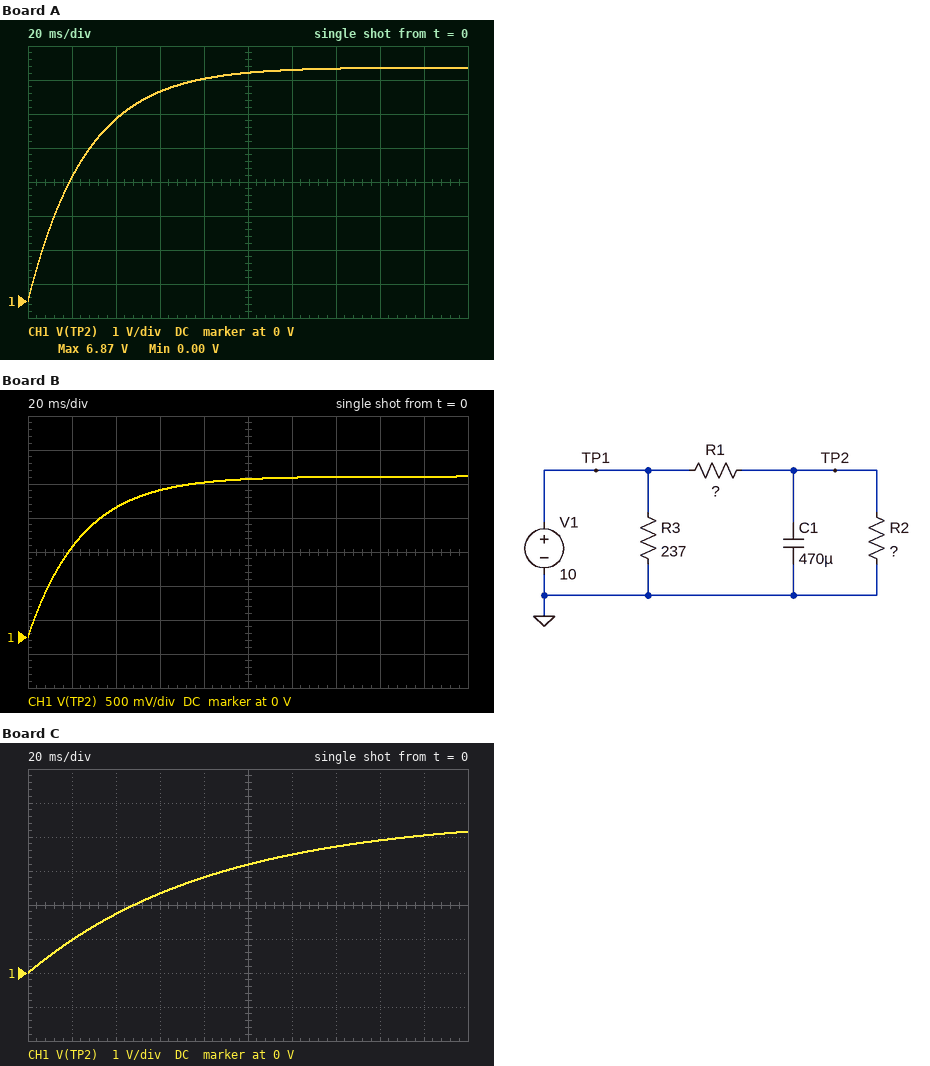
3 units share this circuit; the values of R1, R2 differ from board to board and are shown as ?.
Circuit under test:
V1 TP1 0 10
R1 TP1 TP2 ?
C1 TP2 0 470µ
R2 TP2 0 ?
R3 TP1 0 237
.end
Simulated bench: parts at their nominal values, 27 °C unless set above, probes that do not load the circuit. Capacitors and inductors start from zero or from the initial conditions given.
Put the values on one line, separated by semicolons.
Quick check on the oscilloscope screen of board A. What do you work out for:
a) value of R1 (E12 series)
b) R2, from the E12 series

82 Ω; 180 Ω
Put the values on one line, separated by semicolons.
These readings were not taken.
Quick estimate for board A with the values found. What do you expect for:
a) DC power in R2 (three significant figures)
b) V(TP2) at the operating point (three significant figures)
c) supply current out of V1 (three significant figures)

262 mW; 6.87 V; 80.4 mA
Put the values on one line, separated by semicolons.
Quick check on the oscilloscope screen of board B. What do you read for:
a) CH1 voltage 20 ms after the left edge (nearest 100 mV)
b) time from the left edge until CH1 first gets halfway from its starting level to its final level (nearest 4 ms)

1.3 V; 16 ms
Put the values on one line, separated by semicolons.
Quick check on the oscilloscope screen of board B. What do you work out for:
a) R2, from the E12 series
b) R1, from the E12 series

68 Ω; 220 Ω
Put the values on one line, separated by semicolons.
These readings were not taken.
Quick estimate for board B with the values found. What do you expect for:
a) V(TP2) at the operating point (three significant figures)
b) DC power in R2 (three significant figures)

2.36 V; 82.0 mW
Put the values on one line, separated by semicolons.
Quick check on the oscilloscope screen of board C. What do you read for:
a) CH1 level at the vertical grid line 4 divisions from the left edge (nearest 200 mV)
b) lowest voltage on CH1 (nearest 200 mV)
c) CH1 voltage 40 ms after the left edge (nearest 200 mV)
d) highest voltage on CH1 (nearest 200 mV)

2.8 V; 0 V; 1.8 V; 4.2 V
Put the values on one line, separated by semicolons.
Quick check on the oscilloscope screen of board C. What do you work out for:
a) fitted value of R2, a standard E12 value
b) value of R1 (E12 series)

330 Ω; 390 Ω
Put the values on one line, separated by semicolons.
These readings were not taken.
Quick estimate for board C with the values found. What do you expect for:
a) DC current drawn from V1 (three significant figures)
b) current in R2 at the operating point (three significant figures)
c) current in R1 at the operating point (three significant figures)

56.1 mA; 13.9 mA; 13.9 mA
